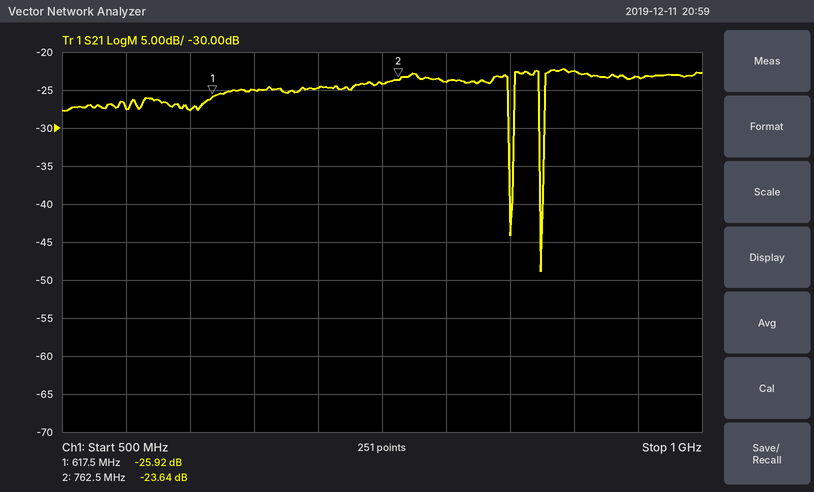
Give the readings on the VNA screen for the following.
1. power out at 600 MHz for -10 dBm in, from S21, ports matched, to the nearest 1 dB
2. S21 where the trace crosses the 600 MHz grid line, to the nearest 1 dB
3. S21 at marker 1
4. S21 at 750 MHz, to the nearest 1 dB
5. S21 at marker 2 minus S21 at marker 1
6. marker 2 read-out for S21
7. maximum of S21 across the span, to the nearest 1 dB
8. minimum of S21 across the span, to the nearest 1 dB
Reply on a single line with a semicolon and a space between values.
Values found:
-38 dBm; -28 dB; -25.92 dB; -24 dB; 2.28 dB; -23.64 dB; -22 dB; -49 dB
